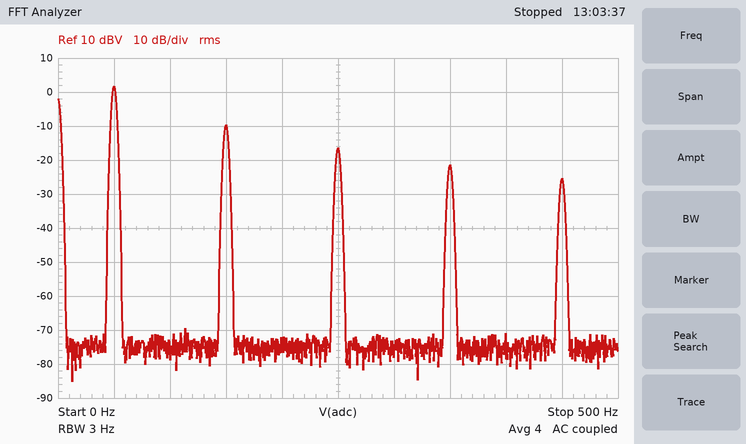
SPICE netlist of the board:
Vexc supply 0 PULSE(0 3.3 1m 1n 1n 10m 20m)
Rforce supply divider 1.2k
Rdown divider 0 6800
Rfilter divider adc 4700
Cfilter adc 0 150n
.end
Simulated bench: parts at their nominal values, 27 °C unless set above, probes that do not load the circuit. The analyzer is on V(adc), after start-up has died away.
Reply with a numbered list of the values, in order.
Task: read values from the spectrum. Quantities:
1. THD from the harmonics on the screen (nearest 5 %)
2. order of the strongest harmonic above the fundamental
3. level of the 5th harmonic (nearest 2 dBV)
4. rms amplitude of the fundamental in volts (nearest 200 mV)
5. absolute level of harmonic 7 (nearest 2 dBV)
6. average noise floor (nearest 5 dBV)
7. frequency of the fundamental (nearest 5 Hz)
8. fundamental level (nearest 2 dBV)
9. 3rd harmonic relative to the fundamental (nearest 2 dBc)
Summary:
1. 30 %
2. 3
3. -16 dBV
4. 1.2 V
5. -22 dBV
6. -75 dBV
7. 50 Hz
8. 2 dBV
9. -12 dBc
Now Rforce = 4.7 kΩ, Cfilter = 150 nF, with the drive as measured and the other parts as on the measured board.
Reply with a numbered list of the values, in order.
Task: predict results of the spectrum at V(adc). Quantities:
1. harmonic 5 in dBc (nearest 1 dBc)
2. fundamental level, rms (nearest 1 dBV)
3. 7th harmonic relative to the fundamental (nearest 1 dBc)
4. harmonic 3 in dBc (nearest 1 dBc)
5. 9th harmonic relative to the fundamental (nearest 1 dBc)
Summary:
1. -20 dBc
2. -2 dBV
3. -25 dBc
4. -12 dBc
5. -29 dBc
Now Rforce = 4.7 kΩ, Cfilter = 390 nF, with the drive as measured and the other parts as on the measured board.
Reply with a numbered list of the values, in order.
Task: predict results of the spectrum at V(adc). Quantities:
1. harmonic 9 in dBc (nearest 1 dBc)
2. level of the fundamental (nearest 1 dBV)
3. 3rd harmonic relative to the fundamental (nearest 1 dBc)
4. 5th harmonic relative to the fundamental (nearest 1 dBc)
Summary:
1. -35 dBc
2. -4 dBV
3. -16 dBc
4. -25 dBc
